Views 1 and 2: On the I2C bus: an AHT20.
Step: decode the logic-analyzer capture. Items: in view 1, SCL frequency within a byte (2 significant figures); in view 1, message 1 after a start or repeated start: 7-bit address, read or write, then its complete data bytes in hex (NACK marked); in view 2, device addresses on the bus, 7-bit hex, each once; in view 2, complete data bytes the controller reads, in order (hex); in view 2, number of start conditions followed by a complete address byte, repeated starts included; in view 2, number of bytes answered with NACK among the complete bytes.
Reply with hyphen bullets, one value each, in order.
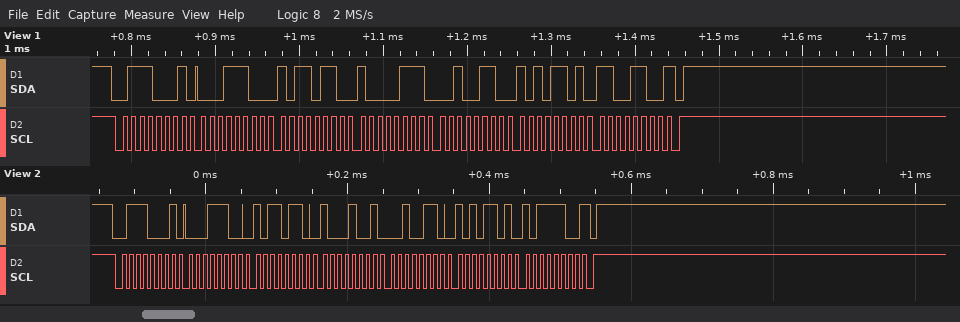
- 100 kHz
- 0x38 read: 1C B6 87 26 AD CC NACK
- 0x38
- 1C B6 89 26 AD BC
- 1
- 1
